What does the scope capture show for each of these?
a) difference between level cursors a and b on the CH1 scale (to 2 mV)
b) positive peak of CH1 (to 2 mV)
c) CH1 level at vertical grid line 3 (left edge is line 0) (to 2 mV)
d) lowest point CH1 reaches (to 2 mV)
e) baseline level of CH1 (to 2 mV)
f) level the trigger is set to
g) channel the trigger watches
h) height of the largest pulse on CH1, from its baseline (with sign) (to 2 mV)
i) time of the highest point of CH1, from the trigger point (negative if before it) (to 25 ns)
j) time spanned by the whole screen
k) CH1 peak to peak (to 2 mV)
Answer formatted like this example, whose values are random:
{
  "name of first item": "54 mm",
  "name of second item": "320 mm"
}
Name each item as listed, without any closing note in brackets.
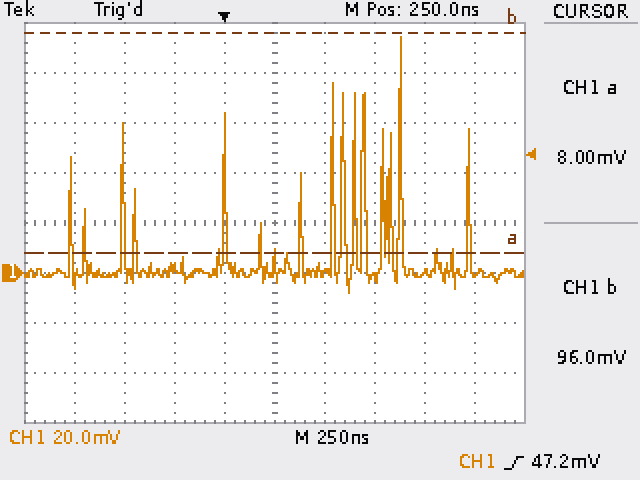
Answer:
{
  "difference between level cursors a and b on the CH1 scale": "88 mV",
  "positive peak of CH1": "94 mV",
  "CH1 level at vertical grid line 3 (left edge is line 0)": "2 mV",
  "lowest point CH1 reaches": "-8 mV",
  "baseline level of CH1": "0 mV",
  "level the trigger is set to": "47.2 mV",
  "channel the trigger watches": "CH1",
  "height of the largest pulse on CH1, from its baseline (with sign)": "+94 mV",
  "time of the highest point of CH1, from the trigger point (negative if before it)": "+875 ns",
  "time spanned by the whole screen": "2.5 µs",
  "CH1 peak to peak": "102 mV"
}
